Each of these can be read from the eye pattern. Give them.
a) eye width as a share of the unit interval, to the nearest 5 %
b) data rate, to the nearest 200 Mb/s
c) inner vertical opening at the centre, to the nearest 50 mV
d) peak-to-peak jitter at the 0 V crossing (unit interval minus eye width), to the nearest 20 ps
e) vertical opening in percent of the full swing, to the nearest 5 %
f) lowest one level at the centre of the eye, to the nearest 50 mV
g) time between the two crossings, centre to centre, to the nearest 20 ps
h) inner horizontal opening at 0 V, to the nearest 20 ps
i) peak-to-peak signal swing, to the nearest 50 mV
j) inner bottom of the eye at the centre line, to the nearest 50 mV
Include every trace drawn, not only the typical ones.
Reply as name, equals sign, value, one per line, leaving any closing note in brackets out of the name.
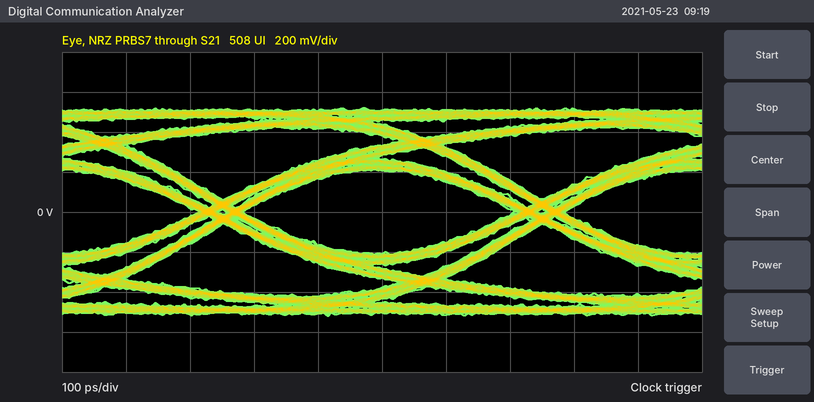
eye width as a share of the unit interval, to the nearest 5 % = 85 %
data rate, to the nearest 200 Mb/s = 2.0 Gb/s
inner vertical opening at the centre, to the nearest 50 mV = 400 mV
peak-to-peak jitter at the 0 V crossing (unit interval minus eye width), to the nearest 20 ps = 80 ps
vertical opening in percent of the full swing, to the nearest 5 % = 40 %
lowest one level at the centre of the eye, to the nearest 50 mV = 200 mV
time between the two crossings, centre to centre, to the nearest 20 ps = 500 ps
inner horizontal opening at 0 V, to the nearest 20 ps = 420 ps
peak-to-peak signal swing, to the nearest 50 mV = 1.05 V
inner bottom of the eye at the centre line, to the nearest 50 mV = -200 mV
